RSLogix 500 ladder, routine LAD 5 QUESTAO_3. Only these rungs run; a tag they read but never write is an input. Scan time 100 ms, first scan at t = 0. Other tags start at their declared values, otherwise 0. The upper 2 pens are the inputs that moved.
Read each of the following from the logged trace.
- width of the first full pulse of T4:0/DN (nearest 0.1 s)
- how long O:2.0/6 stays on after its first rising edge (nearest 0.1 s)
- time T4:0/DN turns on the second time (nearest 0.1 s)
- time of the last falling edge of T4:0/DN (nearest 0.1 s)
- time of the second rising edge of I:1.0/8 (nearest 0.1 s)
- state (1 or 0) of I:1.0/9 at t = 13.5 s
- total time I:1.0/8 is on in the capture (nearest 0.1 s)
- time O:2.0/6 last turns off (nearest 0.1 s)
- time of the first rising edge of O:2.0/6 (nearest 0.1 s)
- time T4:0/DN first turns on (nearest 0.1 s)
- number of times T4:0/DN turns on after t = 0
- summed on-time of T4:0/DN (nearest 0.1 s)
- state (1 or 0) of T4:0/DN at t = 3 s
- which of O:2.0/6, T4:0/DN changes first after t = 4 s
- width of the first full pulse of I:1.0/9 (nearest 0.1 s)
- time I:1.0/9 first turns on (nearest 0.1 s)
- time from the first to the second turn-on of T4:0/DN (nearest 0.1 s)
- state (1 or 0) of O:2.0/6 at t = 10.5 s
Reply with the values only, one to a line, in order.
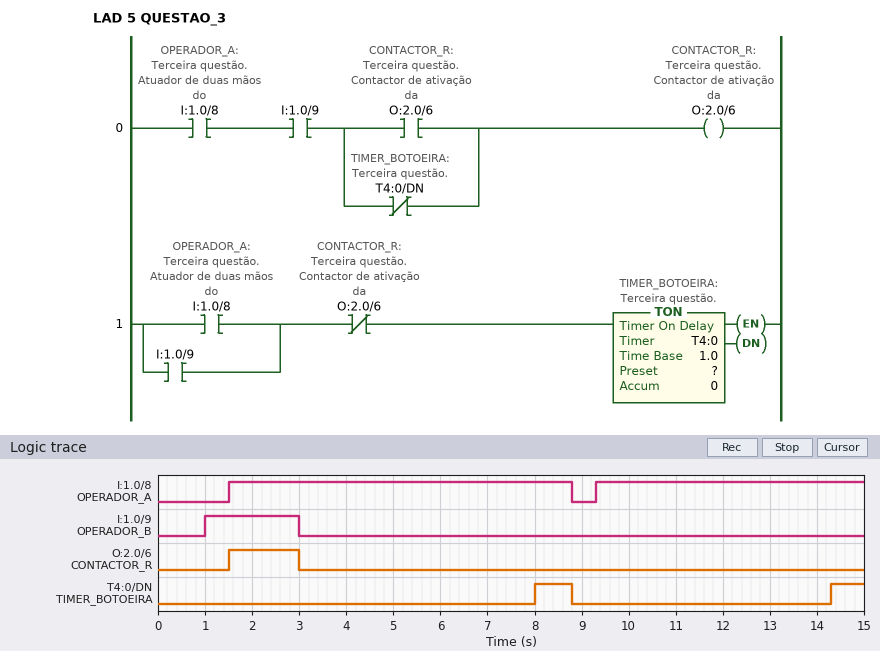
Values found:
0.8 s
1.5 s
14.3 s
8.8 s
9.3 s
0
13.0 s
3.0 s
1.5 s
8.0 s
2
1.5 s
0
T4:0/DN
2.0 s
1.0 s
6.3 s
0
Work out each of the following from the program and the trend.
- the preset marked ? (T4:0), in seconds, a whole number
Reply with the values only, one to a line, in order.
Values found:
5 s
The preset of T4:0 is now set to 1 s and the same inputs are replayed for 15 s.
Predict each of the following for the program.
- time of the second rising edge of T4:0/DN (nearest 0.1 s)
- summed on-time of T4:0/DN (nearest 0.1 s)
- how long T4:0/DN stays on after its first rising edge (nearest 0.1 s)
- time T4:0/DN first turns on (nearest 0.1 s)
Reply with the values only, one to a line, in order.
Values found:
10.3 s
9.5 s
4.8 s
4.0 s
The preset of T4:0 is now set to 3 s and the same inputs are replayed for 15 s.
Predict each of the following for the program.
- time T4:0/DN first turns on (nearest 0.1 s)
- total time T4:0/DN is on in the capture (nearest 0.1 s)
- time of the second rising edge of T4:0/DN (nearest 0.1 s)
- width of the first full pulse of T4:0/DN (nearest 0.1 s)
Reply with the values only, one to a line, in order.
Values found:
6.0 s
5.5 s
12.3 s
2.8 s
